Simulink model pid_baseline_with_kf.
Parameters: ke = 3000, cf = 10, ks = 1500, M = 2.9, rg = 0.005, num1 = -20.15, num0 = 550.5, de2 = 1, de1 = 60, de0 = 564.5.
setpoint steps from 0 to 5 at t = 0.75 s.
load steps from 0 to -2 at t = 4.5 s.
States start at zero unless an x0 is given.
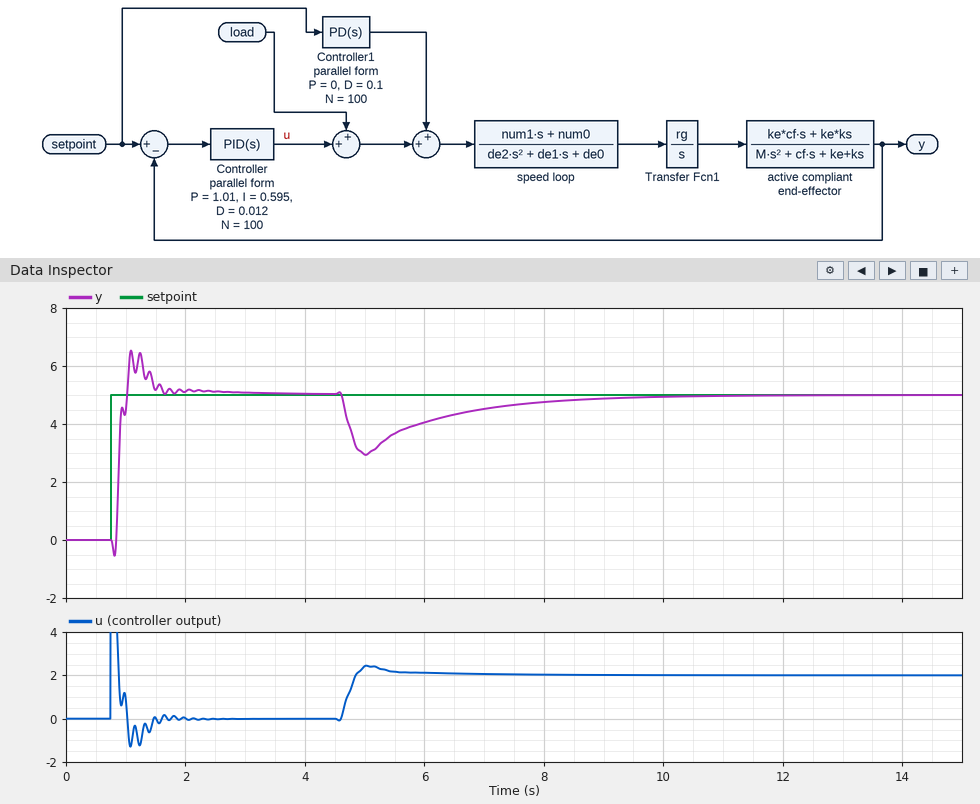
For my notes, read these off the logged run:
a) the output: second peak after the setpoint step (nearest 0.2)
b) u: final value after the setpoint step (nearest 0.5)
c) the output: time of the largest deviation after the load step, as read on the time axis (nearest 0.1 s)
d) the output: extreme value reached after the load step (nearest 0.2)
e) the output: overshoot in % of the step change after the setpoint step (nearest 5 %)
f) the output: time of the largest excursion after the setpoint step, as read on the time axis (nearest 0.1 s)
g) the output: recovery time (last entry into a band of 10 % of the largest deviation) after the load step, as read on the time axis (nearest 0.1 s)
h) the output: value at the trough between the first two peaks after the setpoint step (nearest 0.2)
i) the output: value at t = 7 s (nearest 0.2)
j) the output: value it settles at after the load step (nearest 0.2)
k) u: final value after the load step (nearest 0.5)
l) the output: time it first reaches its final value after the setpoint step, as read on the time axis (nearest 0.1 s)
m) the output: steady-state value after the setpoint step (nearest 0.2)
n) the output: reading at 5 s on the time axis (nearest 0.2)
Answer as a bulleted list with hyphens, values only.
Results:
- 6.4
- 0.0
- 5.0 s
- 3.0
- 30 %
- 1.1 s
- 8.2 s
- 5.8
- 4.6
- 5.0
- 2.0
- 1.0 s
- 5.0
- 3.0
